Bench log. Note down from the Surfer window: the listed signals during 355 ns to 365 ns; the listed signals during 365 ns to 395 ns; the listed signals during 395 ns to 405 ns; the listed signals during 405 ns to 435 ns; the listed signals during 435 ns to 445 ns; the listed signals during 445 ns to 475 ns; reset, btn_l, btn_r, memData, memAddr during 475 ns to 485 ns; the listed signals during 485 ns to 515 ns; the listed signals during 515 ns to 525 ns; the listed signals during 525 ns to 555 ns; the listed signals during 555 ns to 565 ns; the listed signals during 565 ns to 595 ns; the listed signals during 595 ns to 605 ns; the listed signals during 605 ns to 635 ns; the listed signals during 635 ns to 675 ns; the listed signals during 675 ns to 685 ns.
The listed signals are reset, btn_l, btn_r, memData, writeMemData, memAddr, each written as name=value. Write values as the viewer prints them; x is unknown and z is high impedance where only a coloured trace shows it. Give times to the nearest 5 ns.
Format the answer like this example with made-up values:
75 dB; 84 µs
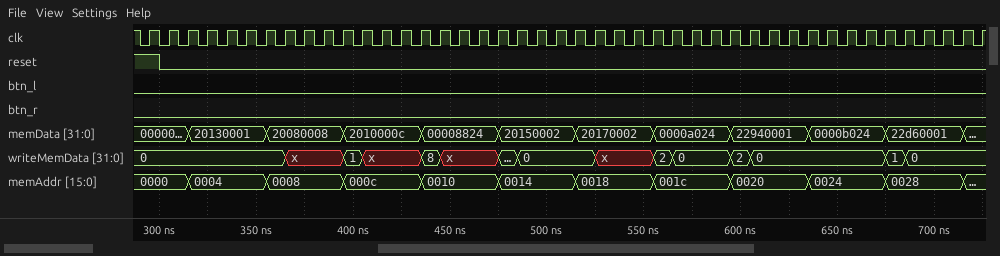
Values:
reset=0, btn_l=0, btn_r=0, memData=20080008, writeMemData=0, memAddr=0008; reset=0, btn_l=0, btn_r=0, memData=20080008, writeMemData=x, memAddr=0008; reset=0, btn_l=0, btn_r=0, memData=2010000c, writeMemData=1, memAddr=000c; reset=0, btn_l=0, btn_r=0, memData=2010000c, writeMemData=x, memAddr=000c; reset=0, btn_l=0, btn_r=0, memData=00008824, writeMemData=8, memAddr=0010; reset=0, btn_l=0, btn_r=0, memData=00008824, writeMemData=x, memAddr=0010; reset=0, btn_l=0, btn_r=0, memData=20150002, memAddr=0014; reset=0, btn_l=0, btn_r=0, memData=20150002, writeMemData=0, memAddr=0014; reset=0, btn_l=0, btn_r=0, memData=20170002, writeMemData=0, memAddr=0018; reset=0, btn_l=0, btn_r=0, memData=20170002, writeMemData=x, memAddr=0018; reset=0, btn_l=0, btn_r=0, memData=0000a024, writeMemData=2, memAddr=001c; reset=0, btn_l=0, btn_r=0, memData=0000a024, writeMemData=0, memAddr=001c; reset=0, btn_l=0, btn_r=0, memData=22940001, writeMemData=2, memAddr=0020; reset=0, btn_l=0, btn_r=0, memData=22940001, writeMemData=0, memAddr=0020; reset=0, btn_l=0, btn_r=0, memData=0000b024, writeMemData=0, memAddr=0024; reset=0, btn_l=0, btn_r=0, memData=22d60001, writeMemData=1, memAddr=0028
